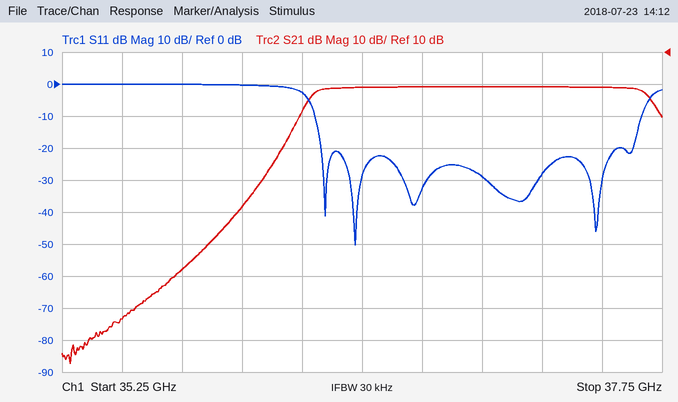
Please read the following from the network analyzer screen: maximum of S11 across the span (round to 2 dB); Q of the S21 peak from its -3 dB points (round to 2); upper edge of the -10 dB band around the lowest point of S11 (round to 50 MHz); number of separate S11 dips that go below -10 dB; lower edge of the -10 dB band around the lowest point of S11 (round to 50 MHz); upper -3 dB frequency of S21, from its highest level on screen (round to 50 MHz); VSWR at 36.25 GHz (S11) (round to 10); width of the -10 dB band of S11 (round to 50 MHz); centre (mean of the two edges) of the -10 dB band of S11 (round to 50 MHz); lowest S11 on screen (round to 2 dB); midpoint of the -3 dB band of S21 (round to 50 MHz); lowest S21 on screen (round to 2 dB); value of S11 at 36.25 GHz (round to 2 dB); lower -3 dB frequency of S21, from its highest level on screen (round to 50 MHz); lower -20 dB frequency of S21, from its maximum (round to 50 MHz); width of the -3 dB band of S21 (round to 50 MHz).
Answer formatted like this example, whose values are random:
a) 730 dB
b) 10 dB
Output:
a) 0 dB
b) 26
c) 37.65 GHz
d) 5
e) 36.30 GHz
f) 37.70 GHz
g) 10
h) 1.35 GHz
i) 37.00 GHz
j) -50 dB
k) 37.00 GHz
l) -88 dB
m) -2 dB
n) 36.30 GHz
o) 36.15 GHz
p) 1.40 GHz
